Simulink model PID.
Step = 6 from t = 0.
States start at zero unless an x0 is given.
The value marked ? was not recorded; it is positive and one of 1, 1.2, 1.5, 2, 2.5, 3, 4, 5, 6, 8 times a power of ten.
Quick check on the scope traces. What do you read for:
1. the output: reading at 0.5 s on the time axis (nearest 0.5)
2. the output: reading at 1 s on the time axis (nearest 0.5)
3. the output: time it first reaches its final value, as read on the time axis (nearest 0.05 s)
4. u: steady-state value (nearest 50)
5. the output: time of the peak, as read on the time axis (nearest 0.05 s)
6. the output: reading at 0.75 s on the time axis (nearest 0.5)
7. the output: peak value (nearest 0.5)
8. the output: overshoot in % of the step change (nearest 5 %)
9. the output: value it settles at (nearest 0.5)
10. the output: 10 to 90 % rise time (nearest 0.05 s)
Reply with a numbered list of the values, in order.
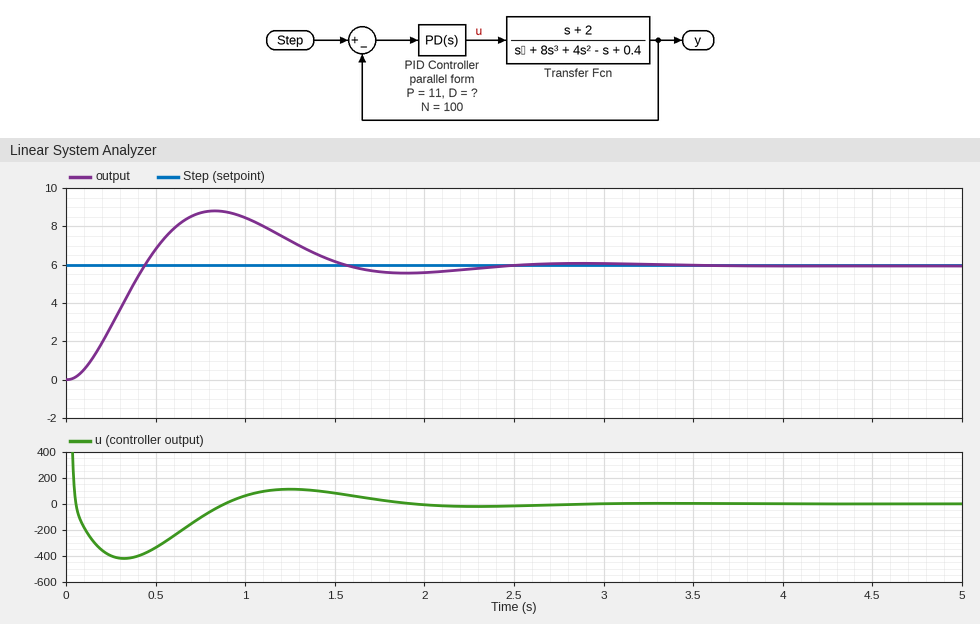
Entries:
1. 7.0
2. 8.5
3. 0.45 s
4. 0
5. 0.85 s
6. 8.5
7. 9.0
8. 50 %
9. 6.0
10. 0.30 s
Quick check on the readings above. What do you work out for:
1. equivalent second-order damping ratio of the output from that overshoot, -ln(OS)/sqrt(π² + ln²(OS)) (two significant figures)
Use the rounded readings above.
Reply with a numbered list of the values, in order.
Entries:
1. 0.22
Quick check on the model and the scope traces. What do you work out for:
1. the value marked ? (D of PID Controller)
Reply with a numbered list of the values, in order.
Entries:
1. 25
